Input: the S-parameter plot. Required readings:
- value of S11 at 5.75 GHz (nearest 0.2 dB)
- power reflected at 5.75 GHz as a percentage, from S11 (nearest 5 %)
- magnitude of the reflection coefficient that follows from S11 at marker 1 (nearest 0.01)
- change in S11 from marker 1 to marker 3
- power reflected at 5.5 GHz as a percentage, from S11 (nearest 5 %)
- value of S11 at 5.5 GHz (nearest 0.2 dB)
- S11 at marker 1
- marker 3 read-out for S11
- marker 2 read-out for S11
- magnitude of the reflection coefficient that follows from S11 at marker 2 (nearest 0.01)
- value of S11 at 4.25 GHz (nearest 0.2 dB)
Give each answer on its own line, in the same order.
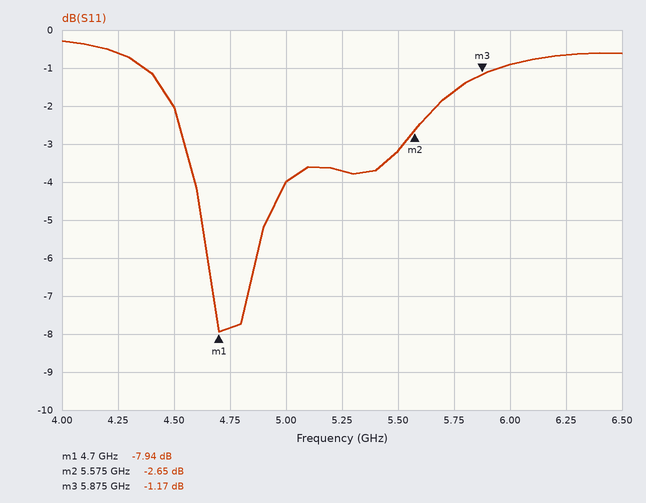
-1.6 dB
70 %
0.40
6.77 dB
50 %
-3.2 dB
-7.94 dB
-1.17 dB
-2.65 dB
0.74
-0.6 dB
